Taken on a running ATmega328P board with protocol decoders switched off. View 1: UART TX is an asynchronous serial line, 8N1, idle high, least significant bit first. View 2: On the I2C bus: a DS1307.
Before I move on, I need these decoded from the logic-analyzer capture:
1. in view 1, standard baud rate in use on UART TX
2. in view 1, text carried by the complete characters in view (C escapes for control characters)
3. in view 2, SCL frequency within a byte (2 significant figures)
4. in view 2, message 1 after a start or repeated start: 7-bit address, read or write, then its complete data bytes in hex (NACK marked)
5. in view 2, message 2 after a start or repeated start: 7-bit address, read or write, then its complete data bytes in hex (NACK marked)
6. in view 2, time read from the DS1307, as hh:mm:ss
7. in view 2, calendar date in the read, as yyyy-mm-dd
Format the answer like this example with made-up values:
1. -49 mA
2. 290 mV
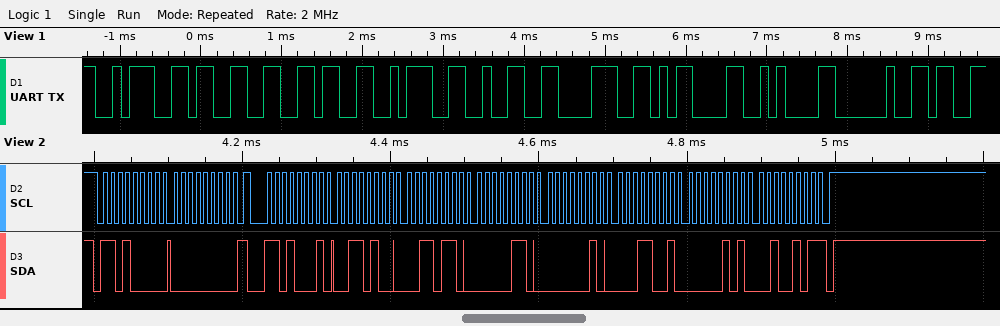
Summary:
1. 9600 baud
2. ":36:28\r\n "
3. 100 kHz
4. 0x68 write: 00
5. 0x68 read: 34 36 06 02 19 05 25 NACK
6. 06:36:34
7. 2025-05-19
